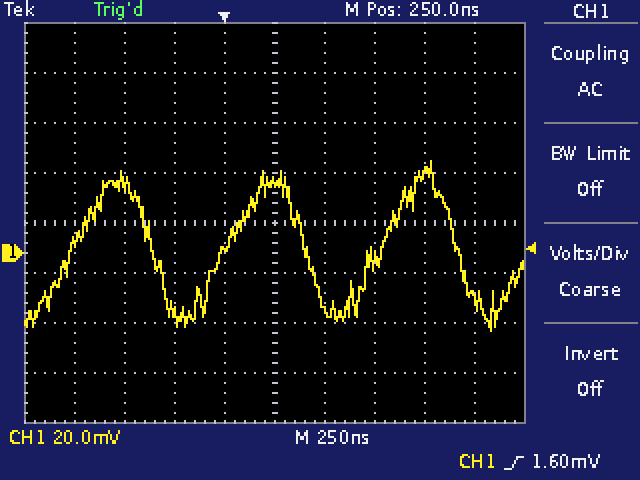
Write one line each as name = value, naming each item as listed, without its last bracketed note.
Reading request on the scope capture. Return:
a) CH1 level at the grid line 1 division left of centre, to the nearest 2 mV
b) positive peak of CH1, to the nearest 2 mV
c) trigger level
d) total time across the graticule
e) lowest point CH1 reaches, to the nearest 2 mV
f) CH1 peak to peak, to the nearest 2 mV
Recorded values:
CH1 level at the grid line 1 division left of centre, to the nearest 2 mV = 2 mV
positive peak of CH1, to the nearest 2 mV = 36 mV
trigger level = 1.60 mV
total time across the graticule = 2.5 µs
lowest point CH1 reaches, to the nearest 2 mV = -32 mV
CH1 peak to peak, to the nearest 2 mV = 68 mV
